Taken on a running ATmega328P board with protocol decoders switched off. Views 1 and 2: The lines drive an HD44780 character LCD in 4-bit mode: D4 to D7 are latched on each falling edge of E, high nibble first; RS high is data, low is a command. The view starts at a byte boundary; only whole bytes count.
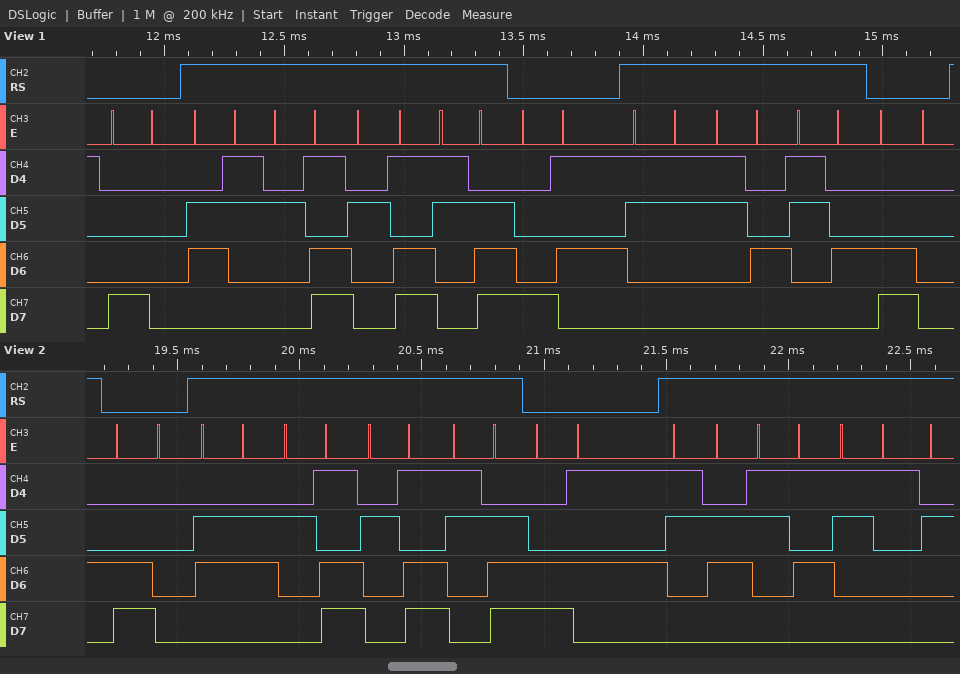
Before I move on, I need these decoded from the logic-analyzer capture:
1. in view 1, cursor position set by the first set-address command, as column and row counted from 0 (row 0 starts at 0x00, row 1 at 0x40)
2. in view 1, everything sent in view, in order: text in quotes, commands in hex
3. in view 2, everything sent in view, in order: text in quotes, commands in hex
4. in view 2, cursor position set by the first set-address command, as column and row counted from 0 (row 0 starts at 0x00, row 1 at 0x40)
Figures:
column 0, row 0
0x80 "c-->" 0x85 "344" 0xC0
0xC0 "f-->" 0xC5 "651"
column 0, row 1
